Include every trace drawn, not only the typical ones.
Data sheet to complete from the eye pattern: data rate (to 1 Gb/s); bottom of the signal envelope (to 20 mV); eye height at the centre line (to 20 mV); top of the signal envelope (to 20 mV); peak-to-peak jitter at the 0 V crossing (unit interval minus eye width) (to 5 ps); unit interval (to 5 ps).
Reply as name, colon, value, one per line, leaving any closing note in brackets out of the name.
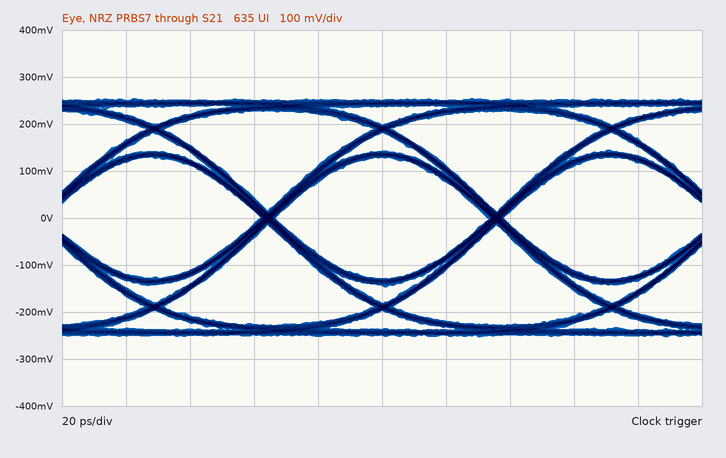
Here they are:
data rate: 14 Gb/s
bottom of the signal envelope: -260 mV
eye height at the centre line: 260 mV
top of the signal envelope: 260 mV
peak-to-peak jitter at the 0 V crossing (unit interval minus eye width): 5 ps
unit interval: 70 ps
